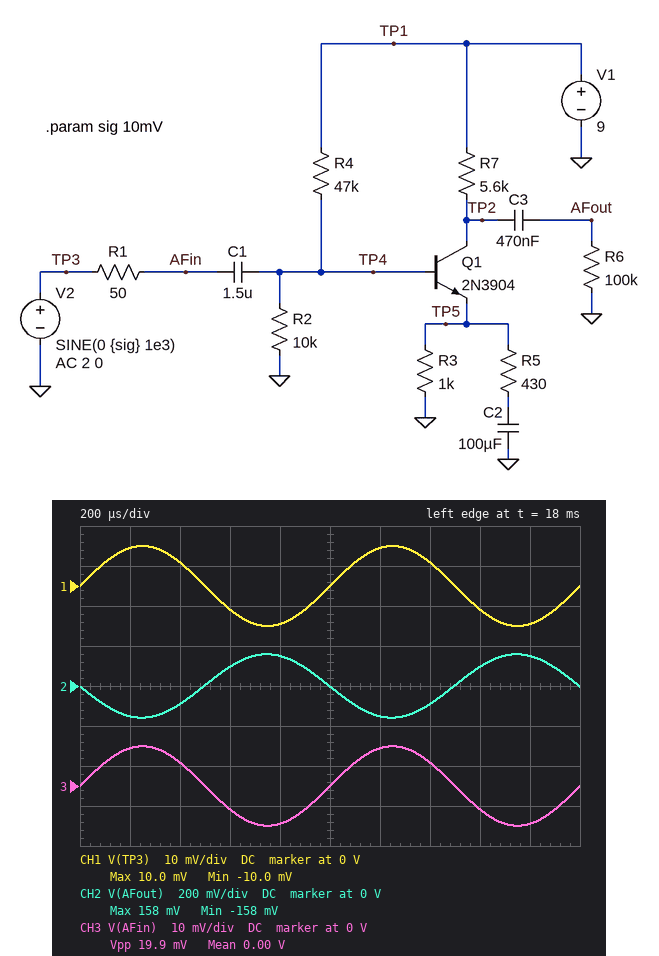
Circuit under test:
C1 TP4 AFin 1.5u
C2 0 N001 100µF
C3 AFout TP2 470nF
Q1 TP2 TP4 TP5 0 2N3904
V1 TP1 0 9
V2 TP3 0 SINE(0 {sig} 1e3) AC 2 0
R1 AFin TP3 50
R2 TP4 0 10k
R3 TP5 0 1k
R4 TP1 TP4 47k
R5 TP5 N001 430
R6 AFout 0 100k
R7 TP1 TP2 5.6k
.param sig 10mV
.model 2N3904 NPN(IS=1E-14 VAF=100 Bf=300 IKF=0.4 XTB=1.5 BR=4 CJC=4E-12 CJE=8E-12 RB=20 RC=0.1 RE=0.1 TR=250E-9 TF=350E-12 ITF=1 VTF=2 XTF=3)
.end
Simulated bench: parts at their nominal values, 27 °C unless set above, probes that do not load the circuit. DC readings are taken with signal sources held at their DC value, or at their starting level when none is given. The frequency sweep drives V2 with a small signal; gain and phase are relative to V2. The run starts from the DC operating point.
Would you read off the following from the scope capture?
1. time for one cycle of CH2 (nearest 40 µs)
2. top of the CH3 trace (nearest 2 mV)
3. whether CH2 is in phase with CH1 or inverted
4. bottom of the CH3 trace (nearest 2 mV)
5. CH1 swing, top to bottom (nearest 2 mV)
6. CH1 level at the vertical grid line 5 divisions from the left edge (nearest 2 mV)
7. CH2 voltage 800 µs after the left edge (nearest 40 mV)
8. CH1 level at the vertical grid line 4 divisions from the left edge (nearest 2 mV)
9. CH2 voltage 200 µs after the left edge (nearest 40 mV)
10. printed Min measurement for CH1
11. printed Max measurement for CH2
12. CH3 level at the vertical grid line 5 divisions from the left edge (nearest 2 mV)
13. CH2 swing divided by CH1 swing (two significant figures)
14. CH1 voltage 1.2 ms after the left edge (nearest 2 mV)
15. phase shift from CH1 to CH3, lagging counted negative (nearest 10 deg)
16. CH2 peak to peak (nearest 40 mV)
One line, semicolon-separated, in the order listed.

1.00 ms; 10 mV; inverted; -10 mV; 20 mV; 0 V; 160 mV; -10 mV; -160 mV; -10.0 mV; 158 mV; 0 V; 16; 10 mV; 0 deg; 320 mV
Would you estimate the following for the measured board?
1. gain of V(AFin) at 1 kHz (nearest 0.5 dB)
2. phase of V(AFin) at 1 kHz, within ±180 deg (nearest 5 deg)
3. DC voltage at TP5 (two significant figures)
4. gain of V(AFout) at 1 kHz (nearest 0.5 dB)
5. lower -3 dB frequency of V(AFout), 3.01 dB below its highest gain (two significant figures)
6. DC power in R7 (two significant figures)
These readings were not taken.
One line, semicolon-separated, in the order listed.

0 dB; 0 deg; 900 mV; 24.0 dB; 15 Hz; 4.5 mW
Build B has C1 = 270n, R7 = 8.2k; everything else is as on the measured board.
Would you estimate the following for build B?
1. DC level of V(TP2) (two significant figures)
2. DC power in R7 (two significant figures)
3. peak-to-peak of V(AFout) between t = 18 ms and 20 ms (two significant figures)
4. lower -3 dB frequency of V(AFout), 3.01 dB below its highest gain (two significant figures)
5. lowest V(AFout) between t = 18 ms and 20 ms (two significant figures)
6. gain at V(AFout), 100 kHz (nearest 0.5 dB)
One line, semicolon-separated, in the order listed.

1.6 V; 6.6 mW; 450 mV; 78 Hz; -230 mV; 27.0 dB
